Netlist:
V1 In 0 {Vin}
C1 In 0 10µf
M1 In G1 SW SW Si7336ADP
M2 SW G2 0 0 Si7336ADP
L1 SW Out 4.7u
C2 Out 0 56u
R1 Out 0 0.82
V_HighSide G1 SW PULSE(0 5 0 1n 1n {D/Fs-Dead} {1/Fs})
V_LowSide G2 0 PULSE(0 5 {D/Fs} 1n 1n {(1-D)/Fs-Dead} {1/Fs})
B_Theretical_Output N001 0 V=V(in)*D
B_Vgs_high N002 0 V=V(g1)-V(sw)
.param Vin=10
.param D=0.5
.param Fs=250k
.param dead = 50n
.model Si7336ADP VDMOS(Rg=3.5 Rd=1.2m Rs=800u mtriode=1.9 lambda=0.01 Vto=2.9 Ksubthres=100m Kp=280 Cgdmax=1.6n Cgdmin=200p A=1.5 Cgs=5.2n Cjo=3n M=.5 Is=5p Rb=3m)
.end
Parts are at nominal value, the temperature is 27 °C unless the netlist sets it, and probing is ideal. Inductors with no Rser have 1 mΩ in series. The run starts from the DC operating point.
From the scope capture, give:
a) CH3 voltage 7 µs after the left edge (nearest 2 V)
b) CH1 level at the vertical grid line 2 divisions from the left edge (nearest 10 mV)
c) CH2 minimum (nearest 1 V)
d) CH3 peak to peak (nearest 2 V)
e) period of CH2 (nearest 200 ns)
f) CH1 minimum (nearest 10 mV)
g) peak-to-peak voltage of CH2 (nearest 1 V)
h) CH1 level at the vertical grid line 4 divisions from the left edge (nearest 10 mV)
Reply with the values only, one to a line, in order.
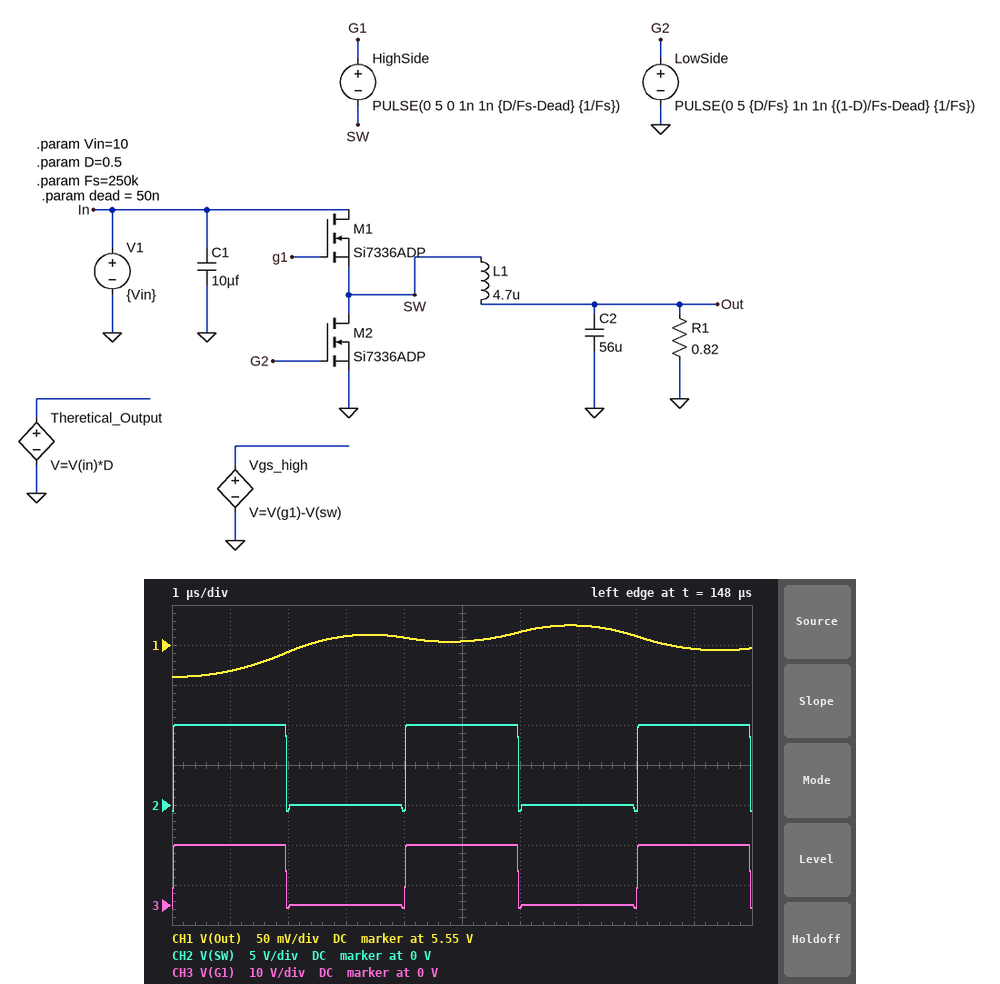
0 V
5.54 V
-1 V
16 V
4.0 µs
5.51 V
11 V
5.56 V
